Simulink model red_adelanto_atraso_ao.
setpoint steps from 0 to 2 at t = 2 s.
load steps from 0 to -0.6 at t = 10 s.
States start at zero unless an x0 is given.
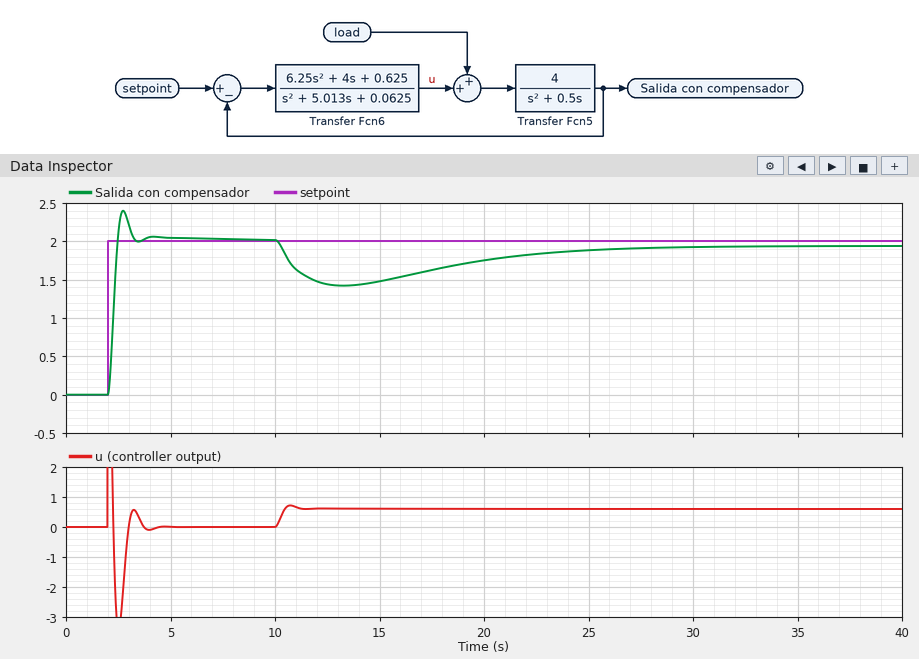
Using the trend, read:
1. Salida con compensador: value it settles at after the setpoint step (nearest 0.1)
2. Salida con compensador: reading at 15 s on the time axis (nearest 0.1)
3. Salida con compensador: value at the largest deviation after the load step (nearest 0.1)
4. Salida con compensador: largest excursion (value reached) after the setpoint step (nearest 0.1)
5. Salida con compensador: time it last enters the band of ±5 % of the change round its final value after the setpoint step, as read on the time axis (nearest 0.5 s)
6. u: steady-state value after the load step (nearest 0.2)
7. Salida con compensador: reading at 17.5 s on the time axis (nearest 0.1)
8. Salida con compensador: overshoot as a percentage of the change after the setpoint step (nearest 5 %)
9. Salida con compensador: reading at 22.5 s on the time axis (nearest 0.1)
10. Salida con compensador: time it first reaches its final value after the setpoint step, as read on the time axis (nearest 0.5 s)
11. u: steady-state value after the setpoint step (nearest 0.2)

2.0
1.5
1.4
2.4
3.0 s
0.6
1.6
20 %
1.8
2.5 s
0.0
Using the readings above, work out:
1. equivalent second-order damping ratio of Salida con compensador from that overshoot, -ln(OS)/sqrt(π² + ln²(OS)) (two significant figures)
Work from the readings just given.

0.46
